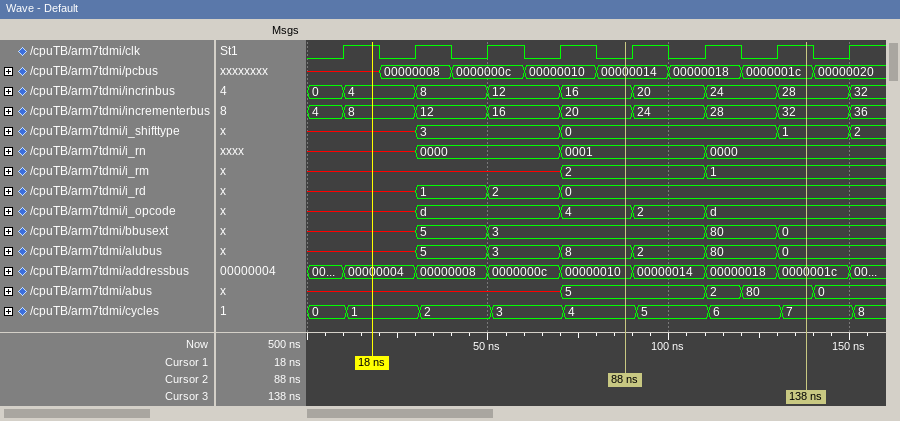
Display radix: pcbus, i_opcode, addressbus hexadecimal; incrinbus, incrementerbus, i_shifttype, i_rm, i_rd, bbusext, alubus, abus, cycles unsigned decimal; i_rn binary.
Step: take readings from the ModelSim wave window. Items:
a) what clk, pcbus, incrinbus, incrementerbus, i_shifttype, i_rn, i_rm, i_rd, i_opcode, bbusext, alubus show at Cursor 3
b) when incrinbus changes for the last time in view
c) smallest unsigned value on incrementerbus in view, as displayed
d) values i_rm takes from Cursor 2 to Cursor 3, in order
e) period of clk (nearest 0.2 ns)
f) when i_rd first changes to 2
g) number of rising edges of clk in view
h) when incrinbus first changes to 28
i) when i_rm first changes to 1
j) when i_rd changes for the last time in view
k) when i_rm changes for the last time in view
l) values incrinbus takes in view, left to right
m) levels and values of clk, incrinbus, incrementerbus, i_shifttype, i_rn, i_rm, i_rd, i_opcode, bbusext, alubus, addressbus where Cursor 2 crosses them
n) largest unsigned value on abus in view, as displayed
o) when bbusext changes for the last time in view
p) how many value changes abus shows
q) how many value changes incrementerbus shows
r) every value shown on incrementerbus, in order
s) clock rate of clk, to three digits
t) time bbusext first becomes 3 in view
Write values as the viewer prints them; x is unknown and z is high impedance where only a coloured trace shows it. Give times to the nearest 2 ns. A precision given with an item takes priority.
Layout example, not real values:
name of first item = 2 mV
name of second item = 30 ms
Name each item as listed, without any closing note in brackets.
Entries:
what clk, pcbus, incrinbus, incrementerbus, i_shifttype, i_rn, i_rm, i_rd, i_opcode, bbusext, alubus show at Cursor 3 = clk=1, pcbus=0000001c, incrinbus=28, incrementerbus=32, i_shifttype=1, i_rn=0000, i_rm=1, i_rd=0, i_opcode=d, bbusext=0, alubus=0
when incrinbus changes for the last time in view = 150 ns
smallest unsigned value on incrementerbus in view, as displayed = 4
values i_rm takes from Cursor 2 to Cursor 3, in order = 2, 1
period of clk = 20 ns
when i_rd first changes to 2 = 50 ns
number of rising edges of clk in view = 8
when incrinbus first changes to 28 = 130 ns
when i_rm first changes to 1 = 110 ns
when i_rd changes for the last time in view = 70 ns
when i_rm changes for the last time in view = 110 ns
values incrinbus takes in view, left to right = 0, 4, 8, 12, 16, 20, 24, 28, 32
levels and values of clk, incrinbus, incrementerbus, i_shifttype, i_rn, i_rm, i_rd, i_opcode, bbusext, alubus, addressbus where Cursor 2 crosses them = clk=0, incrinbus=16, incrementerbus=20, i_shifttype=0, i_rn=0001, i_rm=2, i_rd=0, i_opcode=4, bbusext=3, alubus=8, addressbus=00000010
largest unsigned value on abus in view, as displayed = 80
when bbusext changes for the last time in view = 130 ns
how many value changes abus shows = 4
how many value changes incrementerbus shows = 8
every value shown on incrementerbus, in order = 4, 8, 12, 16, 20, 24, 28, 32, 36
clock rate of clk, to three digits = 50.0 MHz
time bbusext first becomes 3 in view = 50 ns
